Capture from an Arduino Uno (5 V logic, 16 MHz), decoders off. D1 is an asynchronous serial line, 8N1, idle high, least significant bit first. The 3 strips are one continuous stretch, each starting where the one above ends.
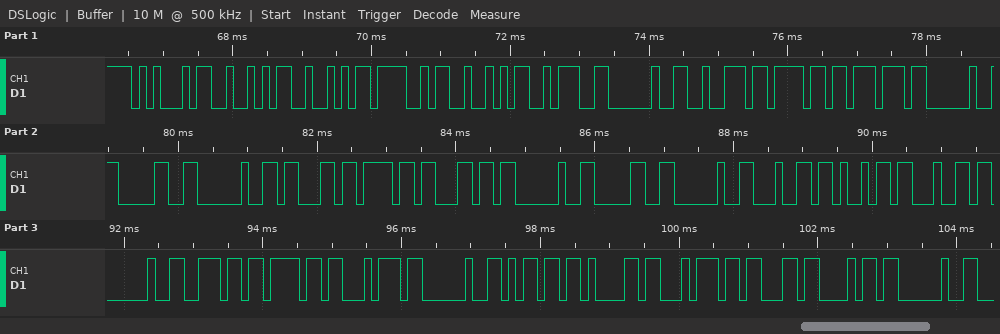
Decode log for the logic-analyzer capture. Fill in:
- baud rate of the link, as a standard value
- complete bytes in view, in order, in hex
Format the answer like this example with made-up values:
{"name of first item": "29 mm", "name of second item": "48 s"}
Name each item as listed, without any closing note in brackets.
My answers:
{"baud rate of the link, as a standard value": "9600 baud", "complete bytes in view, in order, in hex": "45 52 52 4F 52 3A 20 72 6F 77 20 30 20 63 6F 6C 20 30 20 64 69 64 20 6E 6F 74 20 6D 61 74 63 68 20"}
